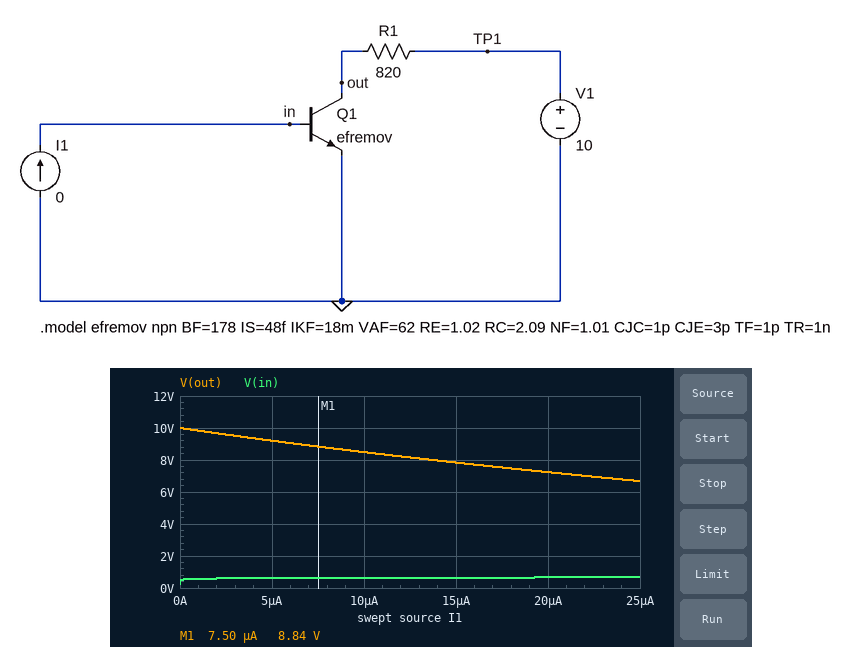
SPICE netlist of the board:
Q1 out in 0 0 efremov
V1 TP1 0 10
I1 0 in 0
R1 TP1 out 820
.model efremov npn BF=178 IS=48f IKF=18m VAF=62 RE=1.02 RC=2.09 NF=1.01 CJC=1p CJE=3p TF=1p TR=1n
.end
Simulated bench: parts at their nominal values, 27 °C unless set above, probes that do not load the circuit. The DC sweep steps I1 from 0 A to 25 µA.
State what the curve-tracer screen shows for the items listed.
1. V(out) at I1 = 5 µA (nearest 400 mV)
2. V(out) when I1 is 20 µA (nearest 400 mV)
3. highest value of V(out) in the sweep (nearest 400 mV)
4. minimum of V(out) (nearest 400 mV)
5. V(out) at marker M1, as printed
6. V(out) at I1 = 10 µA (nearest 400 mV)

9.2 V
7.2 V
10.0 V
6.8 V
8.84 V
8.4 V
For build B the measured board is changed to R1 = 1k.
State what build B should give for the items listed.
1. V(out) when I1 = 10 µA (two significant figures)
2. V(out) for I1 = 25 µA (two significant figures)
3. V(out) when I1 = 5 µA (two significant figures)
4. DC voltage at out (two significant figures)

8.2 V
6.0 V
9.0 V
10 V
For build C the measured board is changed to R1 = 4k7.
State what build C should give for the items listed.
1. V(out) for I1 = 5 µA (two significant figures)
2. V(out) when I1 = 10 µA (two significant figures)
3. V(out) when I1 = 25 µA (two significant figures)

5.7 V
2.1 V
150 mV
